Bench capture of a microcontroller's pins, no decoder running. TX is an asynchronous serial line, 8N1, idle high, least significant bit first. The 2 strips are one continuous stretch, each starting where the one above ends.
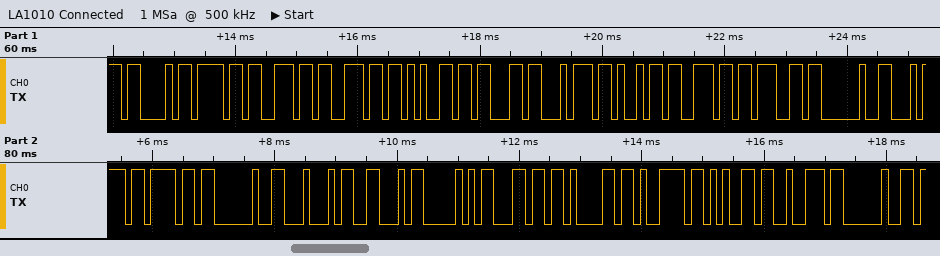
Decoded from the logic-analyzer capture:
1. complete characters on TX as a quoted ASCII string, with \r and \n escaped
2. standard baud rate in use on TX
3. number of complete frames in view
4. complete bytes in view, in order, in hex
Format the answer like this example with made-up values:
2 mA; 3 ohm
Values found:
"Connecting to DFPlayer "; 9600 baud; 23; 43 6F 6E 6E 65 63 74 69 6E 67 20 74 6F 20 44 46 50 6C 61 79 65 72 20
